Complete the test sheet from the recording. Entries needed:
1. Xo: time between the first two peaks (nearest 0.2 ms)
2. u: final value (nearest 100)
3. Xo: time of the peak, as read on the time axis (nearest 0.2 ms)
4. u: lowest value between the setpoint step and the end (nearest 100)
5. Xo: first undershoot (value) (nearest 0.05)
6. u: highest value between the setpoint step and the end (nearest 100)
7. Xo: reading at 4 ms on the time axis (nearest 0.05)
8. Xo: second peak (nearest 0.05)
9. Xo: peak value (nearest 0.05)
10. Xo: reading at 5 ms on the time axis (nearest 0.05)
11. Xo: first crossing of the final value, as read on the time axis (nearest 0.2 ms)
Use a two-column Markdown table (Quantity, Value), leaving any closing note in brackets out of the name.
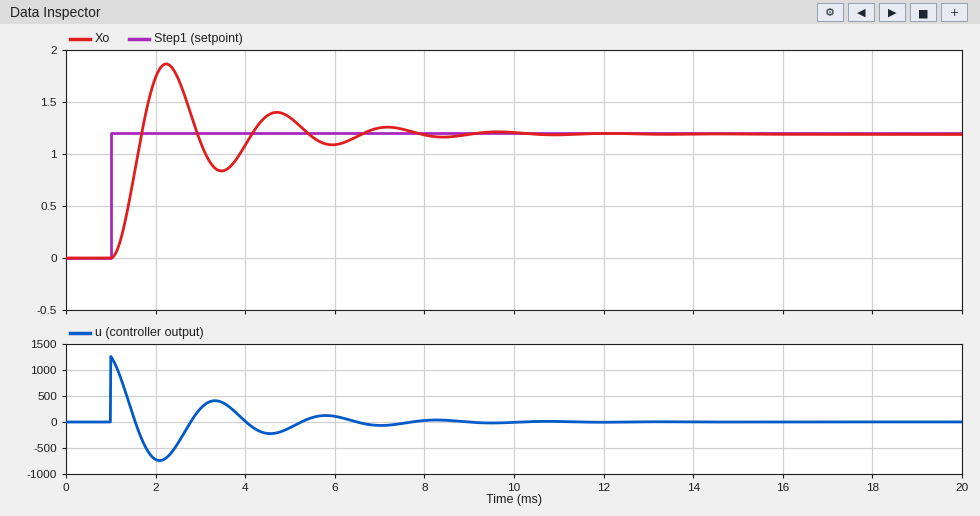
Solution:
| Quantity | Value |
|---|---|
| Xo: time between the first two peaks | 2.4 ms |
| u: final value | 0 |
| Xo: time of the peak, as read on the time axis | 2.2 ms |
| u: lowest value between the setpoint step and the end | -700 |
| Xo: first undershoot (value) | 0.85 |
| u: highest value between the setpoint step and the end | 1300 |
| Xo: reading at 4 ms on the time axis | 1.10 |
| Xo: second peak | 1.40 |
| Xo: peak value | 1.85 |
| Xo: reading at 5 ms on the time axis | 1.35 |
| Xo: first crossing of the final value, as read on the time axis | 1.6 ms |
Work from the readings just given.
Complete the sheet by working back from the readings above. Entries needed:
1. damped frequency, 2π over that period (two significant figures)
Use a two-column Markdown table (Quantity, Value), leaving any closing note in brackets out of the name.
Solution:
| Quantity | Value |
|---|---|
| damped frequency, 2π over that period | 2.6 rad/ms |
